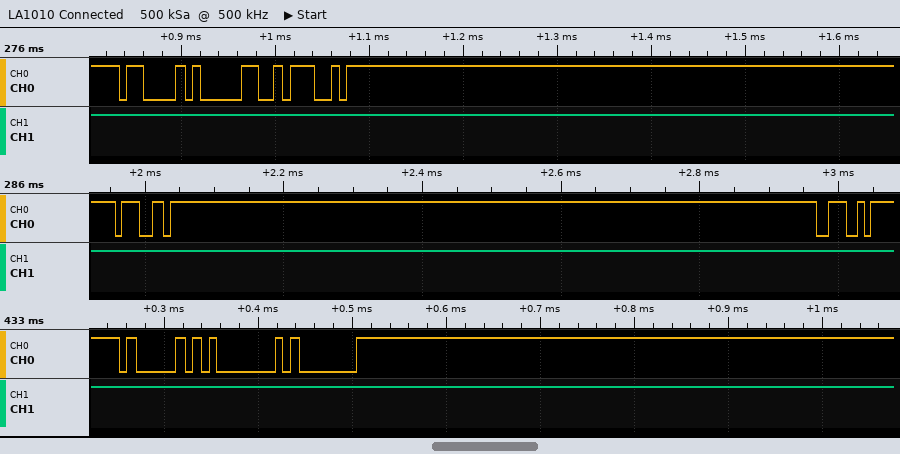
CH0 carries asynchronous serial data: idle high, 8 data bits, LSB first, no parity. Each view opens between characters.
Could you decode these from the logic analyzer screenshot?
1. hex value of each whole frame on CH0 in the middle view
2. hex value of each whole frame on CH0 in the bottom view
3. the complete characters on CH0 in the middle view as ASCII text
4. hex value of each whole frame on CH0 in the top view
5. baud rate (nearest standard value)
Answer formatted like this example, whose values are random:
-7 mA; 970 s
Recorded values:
67, 4E; 41, 01, 01; "gN"; 43, 30, A7; 115200 baud
